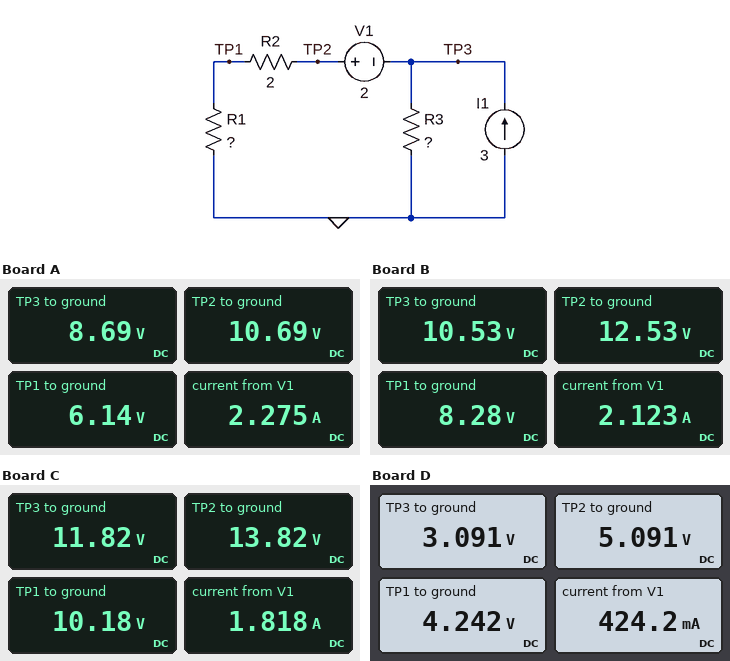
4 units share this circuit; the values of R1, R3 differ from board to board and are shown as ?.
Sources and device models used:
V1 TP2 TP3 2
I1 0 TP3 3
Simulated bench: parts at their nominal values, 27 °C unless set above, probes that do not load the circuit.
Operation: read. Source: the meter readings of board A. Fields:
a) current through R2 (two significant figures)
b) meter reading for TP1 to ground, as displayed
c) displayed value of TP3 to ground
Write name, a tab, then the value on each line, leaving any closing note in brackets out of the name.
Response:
current through R2	2.3 A
meter reading for TP1 to ground, as displayed	6.14 V
displayed value of TP3 to ground	8.69 V
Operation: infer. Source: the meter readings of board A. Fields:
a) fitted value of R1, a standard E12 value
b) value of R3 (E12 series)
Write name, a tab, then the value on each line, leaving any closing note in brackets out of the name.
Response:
fitted value of R1, a standard E12 value	2.7 Ω
value of R3	12 Ω
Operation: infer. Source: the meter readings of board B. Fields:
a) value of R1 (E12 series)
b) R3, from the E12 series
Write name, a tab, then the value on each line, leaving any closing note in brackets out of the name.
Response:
value of R1	3.9 Ω
R3, from the E12 series	12 Ω
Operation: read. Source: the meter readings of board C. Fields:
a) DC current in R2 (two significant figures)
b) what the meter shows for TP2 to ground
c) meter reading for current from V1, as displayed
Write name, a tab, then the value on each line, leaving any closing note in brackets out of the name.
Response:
DC current in R2	1.8 A
what the meter shows for TP2 to ground	13.82 V
meter reading for current from V1, as displayed	1.818 A
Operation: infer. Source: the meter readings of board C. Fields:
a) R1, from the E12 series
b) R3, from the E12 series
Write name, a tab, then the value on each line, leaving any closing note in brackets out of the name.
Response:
R1, from the E12 series	5.6 Ω
R3, from the E12 series	10 Ω
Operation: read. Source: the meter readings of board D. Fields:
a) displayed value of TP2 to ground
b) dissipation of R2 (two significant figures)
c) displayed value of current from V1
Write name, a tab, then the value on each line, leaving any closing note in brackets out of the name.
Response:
displayed value of TP2 to ground	5.091 V
dissipation of R2	360 mW
displayed value of current from V1	424.2 mA
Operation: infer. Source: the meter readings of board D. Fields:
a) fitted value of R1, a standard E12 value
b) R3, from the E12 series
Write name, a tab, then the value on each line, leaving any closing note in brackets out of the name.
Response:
fitted value of R1, a standard E12 value	10 Ω
R3, from the E12 series	1.2 Ω
